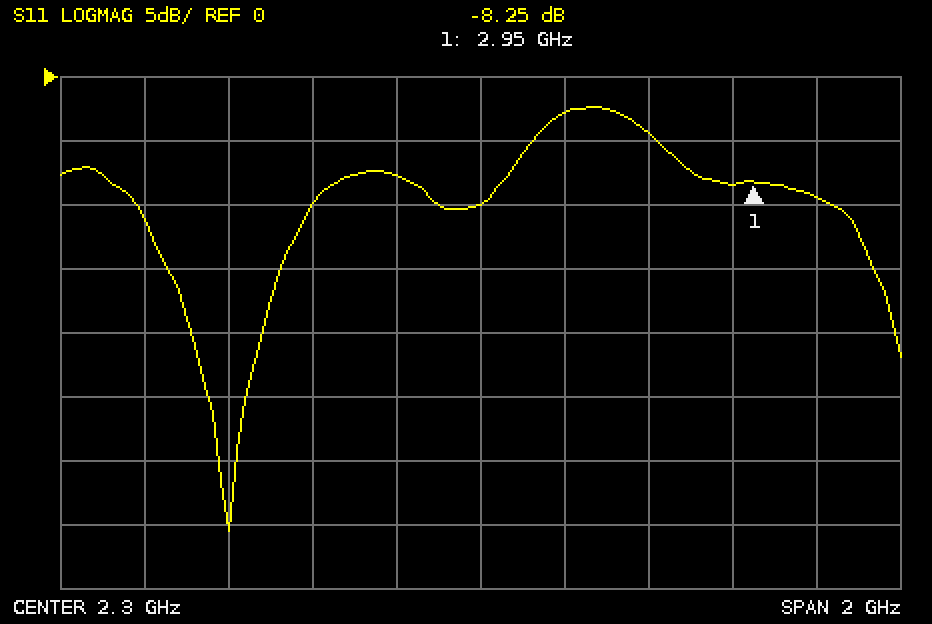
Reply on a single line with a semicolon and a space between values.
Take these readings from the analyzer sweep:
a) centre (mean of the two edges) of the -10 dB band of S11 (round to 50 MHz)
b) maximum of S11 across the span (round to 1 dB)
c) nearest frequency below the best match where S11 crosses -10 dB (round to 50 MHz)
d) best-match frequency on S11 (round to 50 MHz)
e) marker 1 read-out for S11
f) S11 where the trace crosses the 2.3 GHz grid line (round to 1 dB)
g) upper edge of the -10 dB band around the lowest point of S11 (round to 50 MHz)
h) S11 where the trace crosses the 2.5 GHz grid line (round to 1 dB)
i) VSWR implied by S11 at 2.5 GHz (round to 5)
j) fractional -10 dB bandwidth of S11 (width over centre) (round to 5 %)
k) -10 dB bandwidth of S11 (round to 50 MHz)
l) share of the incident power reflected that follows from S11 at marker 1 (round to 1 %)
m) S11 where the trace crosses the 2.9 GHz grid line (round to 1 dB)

1.70 GHz; -2 dB; 1.50 GHz; 1.70 GHz; -8.25 dB; -10 dB; 1.90 GHz; -3 dB; 5; 25 %; 400 MHz; 15 %; -8 dB
